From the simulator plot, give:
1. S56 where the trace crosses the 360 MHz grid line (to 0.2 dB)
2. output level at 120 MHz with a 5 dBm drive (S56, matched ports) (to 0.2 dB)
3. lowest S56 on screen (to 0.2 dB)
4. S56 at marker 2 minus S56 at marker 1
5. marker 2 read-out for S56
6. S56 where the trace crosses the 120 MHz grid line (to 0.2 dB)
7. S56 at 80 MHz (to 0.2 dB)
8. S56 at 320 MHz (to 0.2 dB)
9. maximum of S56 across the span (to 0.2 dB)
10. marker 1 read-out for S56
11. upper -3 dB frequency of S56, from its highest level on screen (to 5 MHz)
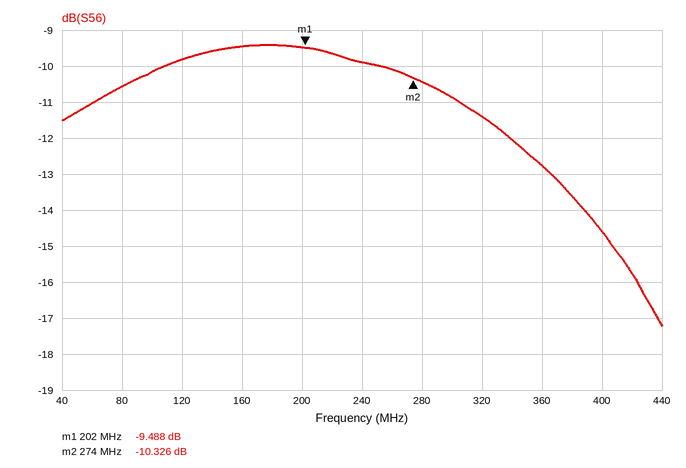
-12.8 dB
-4.8 dBm
-17.2 dB
-0.838 dB
-10.326 dB
-9.8 dB
-10.6 dB
-11.4 dB
-9.4 dB
-9.488 dB
350 MHz
